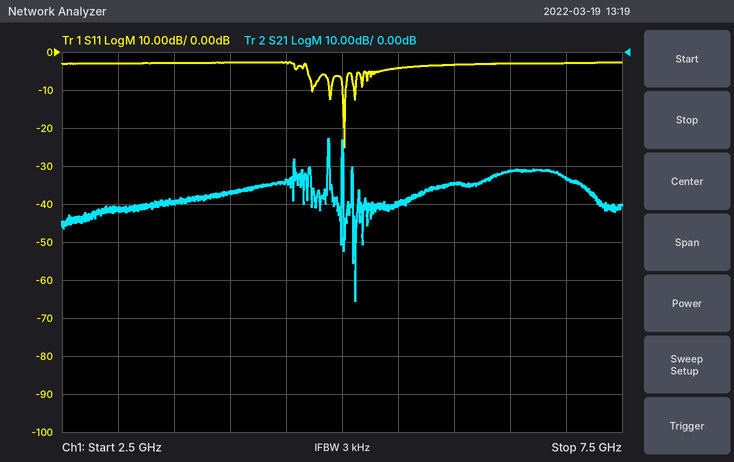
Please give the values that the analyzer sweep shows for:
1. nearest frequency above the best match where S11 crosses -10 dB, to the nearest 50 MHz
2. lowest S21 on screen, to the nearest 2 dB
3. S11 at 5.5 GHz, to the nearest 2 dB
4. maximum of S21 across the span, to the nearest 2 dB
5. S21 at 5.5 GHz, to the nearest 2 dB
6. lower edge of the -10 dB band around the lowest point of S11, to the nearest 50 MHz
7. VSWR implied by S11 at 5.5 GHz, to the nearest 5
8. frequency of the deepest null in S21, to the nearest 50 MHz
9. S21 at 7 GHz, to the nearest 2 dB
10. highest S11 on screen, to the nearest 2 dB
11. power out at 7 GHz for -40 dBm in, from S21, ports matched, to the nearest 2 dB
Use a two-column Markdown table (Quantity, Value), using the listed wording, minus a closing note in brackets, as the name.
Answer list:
| Quantity | Value |
|---|---|
| nearest frequency above the best match where S11 crosses -10 dB, to the nearest 50 MHz | 5.05 GHz |
| lowest S21 on screen, to the nearest 2 dB | -66 dB |
| S11 at 5.5 GHz, to the nearest 2 dB | -4 dB |
| maximum of S21 across the span, to the nearest 2 dB | -22 dB |
| S21 at 5.5 GHz, to the nearest 2 dB | -40 dB |
| lower edge of the -10 dB band around the lowest point of S11, to the nearest 50 MHz | 5.00 GHz |
| VSWR implied by S11 at 5.5 GHz, to the nearest 5 | 5 |
| frequency of the deepest null in S21, to the nearest 50 MHz | 5.10 GHz |
| S21 at 7 GHz, to the nearest 2 dB | -34 dB |
| highest S11 on screen, to the nearest 2 dB | -2 dB |
| power out at 7 GHz for -40 dBm in, from S21, ports matched, to the nearest 2 dB | -74 dBm |
